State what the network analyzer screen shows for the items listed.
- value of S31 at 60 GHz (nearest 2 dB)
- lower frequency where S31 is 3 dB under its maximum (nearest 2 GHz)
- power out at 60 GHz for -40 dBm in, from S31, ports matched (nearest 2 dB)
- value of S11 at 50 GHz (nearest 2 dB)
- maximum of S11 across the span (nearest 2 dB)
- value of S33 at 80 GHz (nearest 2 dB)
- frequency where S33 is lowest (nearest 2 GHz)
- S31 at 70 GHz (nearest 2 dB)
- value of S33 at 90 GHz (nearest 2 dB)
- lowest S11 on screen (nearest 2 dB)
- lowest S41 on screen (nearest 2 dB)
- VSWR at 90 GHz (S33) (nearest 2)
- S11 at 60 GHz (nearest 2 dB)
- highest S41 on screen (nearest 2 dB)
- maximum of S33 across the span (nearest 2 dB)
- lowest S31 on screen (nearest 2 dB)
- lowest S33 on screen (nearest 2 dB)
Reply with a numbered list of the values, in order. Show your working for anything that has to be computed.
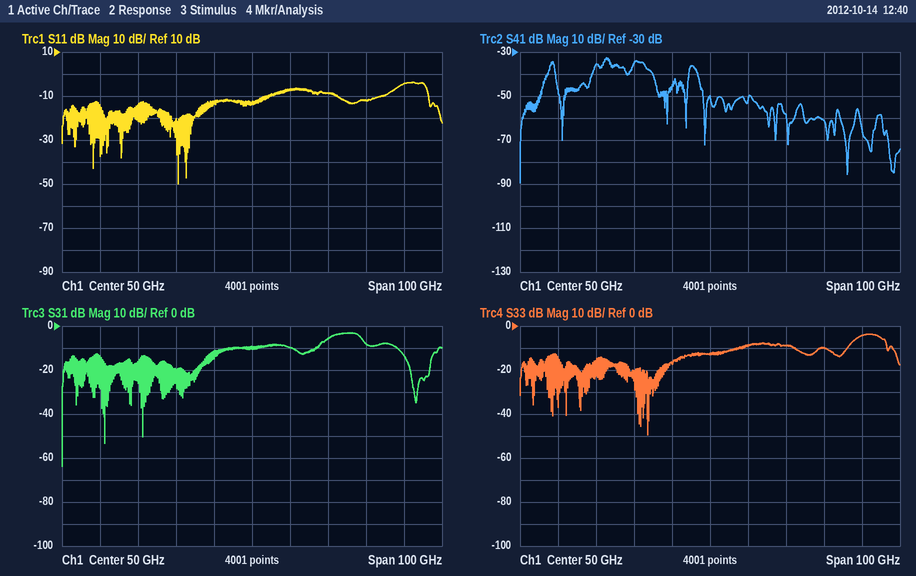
1. -10 dB
2. 70 GHz
3. -40 dBm + (-10 dB) = -50 dBm
4. -14 dB
5. -4 dB
6. -10 dB
7. 34 GHz
8. -6 dB
9. -4 dB
10. -50 dB
11. -90 dB
12. |Γ| = 10^(-4/20) = 0.6310; VSWR = (1 + 0.6310)/(1 − 0.6310) ≈ 4
13. -8 dB
14. -32 dB
15. -4 dB
16. -64 dB
17. -50 dB
